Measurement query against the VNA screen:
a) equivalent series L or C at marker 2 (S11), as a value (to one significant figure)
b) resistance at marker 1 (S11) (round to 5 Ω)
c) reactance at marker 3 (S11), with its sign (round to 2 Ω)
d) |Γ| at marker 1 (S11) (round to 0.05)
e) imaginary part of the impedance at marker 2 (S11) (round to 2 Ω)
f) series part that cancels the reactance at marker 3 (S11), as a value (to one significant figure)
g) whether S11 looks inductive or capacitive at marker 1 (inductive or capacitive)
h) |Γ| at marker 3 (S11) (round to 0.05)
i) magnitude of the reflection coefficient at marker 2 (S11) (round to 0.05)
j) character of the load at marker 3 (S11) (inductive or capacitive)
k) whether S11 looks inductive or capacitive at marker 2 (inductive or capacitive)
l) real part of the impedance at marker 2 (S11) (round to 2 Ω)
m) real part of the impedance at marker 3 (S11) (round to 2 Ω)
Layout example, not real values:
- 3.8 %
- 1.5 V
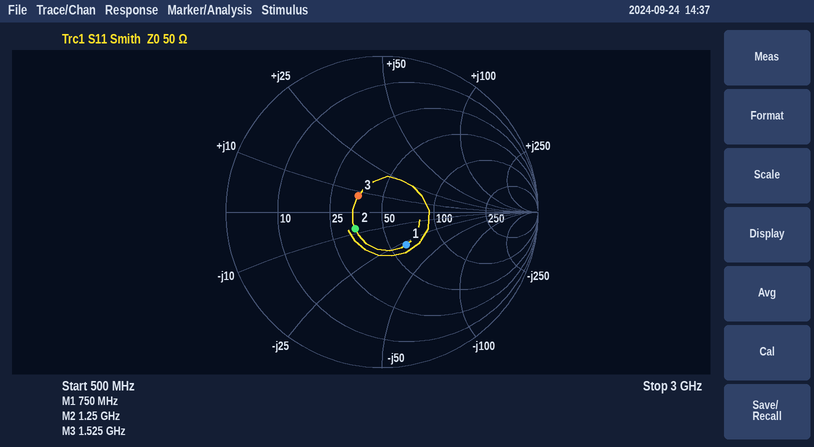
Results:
- 20 pF
- 60 Ω
- +8 Ω
- 0.25
- -8 Ω
- 10 pF
- capacitive
- 0.20
- 0.20
- inductive
- capacitive
- 34 Ω
- 36 Ω
